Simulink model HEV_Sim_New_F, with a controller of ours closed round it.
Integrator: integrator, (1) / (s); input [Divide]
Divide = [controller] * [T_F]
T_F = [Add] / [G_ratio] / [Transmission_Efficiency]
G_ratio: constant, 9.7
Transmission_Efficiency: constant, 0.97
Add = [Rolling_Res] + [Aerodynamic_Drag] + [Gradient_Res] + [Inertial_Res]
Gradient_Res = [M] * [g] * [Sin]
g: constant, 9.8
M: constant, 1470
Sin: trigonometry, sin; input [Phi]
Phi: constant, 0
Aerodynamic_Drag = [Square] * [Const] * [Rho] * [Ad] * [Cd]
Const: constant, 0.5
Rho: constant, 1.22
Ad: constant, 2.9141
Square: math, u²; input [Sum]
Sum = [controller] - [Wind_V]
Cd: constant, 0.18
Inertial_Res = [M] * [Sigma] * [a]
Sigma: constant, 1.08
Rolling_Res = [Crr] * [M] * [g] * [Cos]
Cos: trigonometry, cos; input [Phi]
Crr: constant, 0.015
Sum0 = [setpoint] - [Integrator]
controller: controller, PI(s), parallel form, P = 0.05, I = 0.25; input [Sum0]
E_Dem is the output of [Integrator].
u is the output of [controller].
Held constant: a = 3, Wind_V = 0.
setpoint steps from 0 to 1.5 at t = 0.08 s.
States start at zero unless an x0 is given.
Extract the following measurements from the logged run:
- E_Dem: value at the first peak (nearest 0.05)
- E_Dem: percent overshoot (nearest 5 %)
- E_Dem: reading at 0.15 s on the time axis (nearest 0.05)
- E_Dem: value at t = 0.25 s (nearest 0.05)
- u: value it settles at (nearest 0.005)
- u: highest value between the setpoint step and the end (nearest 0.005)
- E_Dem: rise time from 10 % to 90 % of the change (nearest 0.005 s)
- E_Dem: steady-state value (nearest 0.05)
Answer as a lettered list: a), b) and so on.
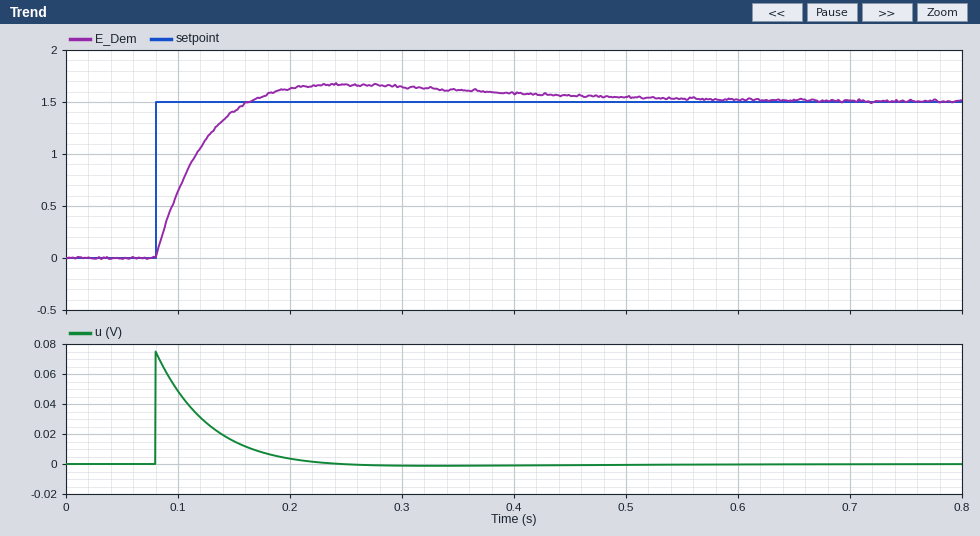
a) 1.65
b) 10 %
c) 1.40
d) 1.65
e) 0.000
f) 0.075
g) 0.060 s
h) 1.50
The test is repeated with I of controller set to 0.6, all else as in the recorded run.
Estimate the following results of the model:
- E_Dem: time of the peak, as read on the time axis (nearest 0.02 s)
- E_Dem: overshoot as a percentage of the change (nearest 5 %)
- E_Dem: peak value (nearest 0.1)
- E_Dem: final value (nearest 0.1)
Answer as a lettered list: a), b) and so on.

a) 0.20 s
b) 20 %
c) 1.8
d) 1.5
